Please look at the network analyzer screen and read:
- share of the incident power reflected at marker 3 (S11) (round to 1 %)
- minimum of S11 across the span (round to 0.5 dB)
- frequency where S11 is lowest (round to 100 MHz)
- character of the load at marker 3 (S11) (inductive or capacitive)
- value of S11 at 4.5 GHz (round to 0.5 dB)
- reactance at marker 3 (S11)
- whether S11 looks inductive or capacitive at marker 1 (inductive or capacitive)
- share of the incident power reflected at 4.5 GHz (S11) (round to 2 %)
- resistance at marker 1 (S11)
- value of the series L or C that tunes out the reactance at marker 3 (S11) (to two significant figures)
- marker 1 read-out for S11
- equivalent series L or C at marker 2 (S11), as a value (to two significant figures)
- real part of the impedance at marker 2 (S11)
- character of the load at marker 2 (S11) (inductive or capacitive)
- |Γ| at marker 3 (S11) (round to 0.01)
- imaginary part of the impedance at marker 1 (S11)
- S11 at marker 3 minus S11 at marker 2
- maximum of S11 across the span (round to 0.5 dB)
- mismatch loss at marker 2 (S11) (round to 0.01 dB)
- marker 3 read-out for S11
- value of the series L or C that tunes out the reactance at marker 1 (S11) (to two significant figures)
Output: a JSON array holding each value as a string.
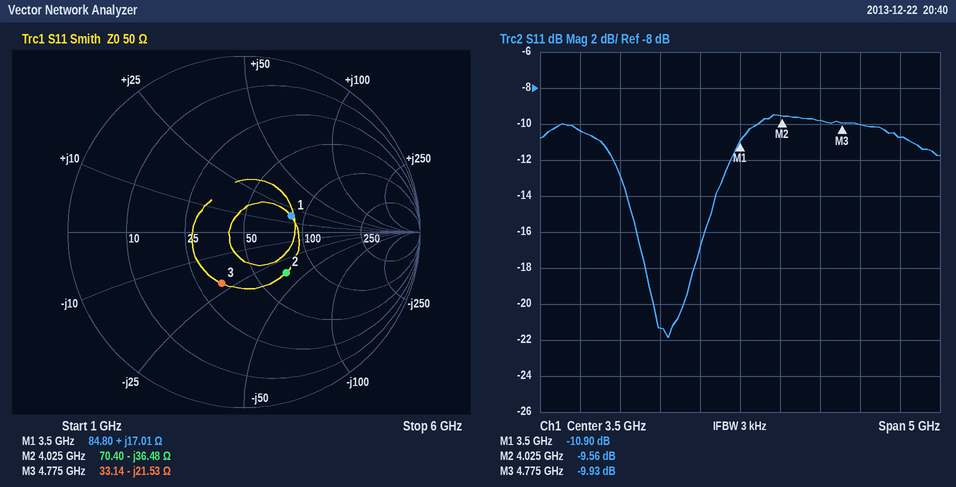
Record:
["10 %", "-22.0 dB", "2.6 GHz", "capacitive", "-10.0 dB", "-21.53 Ω", "inductive", "10 %", "84.80 Ω", "720 pH", "-10.90 dB", "1.1 pF", "70.40 Ω", "capacitive", "0.32", "+17.01 Ω", "-0.37 dB", "-9.5 dB", "0.51 dB", "-9.93 dB", "2.7 pF"]
